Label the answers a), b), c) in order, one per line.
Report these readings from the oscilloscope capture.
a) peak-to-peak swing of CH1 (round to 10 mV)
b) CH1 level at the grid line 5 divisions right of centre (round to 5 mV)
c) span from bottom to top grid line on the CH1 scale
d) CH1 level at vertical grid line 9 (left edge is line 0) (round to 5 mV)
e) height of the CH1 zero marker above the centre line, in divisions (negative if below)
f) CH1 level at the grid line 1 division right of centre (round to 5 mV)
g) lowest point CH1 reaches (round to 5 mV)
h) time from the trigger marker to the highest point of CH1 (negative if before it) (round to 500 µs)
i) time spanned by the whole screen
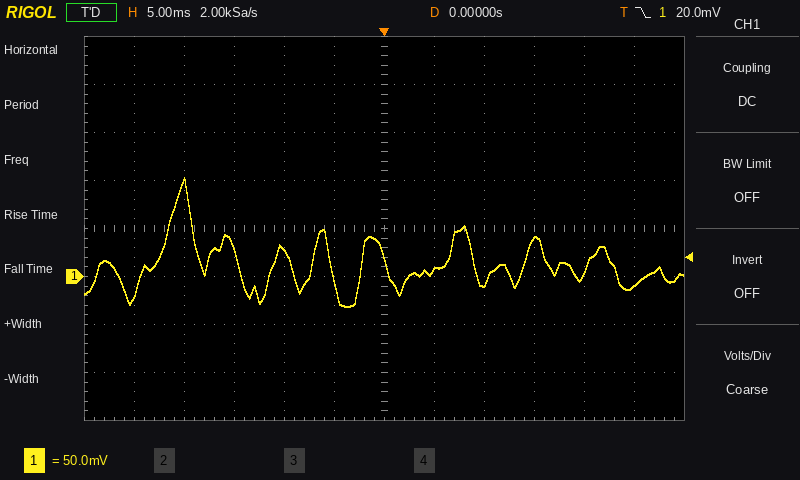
a) 130 mV
b) -10 mV
c) 400 mV
d) 40 mV
e) -1.0 div
f) 5 mV
g) -30 mV
h) -20.0 ms
i) 60 ms
